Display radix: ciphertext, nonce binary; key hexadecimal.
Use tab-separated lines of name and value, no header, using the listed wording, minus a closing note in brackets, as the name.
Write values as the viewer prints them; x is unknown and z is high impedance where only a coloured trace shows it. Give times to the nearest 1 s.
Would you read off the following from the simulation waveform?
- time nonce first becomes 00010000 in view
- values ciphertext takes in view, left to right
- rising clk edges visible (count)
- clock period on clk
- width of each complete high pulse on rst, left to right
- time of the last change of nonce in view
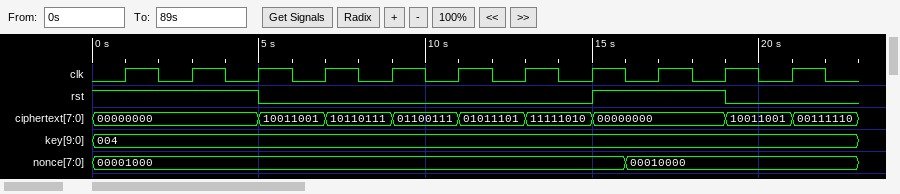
time nonce first becomes 00010000 in view	16 s
values ciphertext takes in view, left to right	00000000, 10011001, 10110111, 01100111, 01011101, 11111010, 00000000, 10011001, 00111110
rising clk edges visible	11
clock period on clk	2 s
width of each complete high pulse on rst, left to right	4 s
time of the last change of nonce in view	16 s
